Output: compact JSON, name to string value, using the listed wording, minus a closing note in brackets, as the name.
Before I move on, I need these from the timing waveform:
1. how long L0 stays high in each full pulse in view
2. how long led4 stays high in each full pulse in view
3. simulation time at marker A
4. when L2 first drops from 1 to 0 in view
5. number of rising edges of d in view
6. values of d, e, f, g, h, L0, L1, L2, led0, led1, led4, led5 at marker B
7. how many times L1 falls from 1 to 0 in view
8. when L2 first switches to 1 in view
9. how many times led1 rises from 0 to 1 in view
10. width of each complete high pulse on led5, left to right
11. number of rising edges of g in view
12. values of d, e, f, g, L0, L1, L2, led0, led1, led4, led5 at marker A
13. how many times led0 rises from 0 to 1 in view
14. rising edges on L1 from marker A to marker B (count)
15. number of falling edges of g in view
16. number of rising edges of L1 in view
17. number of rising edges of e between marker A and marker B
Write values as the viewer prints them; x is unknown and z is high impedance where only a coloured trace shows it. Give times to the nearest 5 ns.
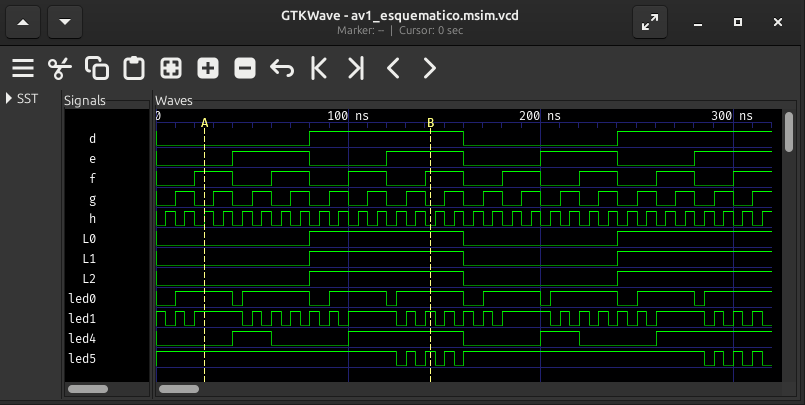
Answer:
{"how long L0 stays high in each full pulse in view": "80 ns", "how long led4 stays high in each full pulse in view": "20 ns, 60 ns, 20 ns", "simulation time at marker A": "25 ns", "when L2 first drops from 1 to 0 in view": "160 ns", "number of rising edges of d in view": "2", "values of d, e, f, g, h, L0, L1, L2, led0, led1, led4, led5 at marker B": "d=1, e=1, f=1, g=0, h=0, L0=1, L1=1, L2=1, led0=1, led1=1, led4=1, led5=1", "how many times L1 falls from 1 to 0 in view": "1", "when L2 first switches to 1 in view": "80 ns", "how many times led1 rises from 0 to 1 in view": "23", "width of each complete high pulse on led5, left to right": "5 ns, 5 ns, 5 ns, 125 ns, 5 ns, 5 ns, 5 ns", "number of rising edges of g in view": "16", "values of d, e, f, g, L0, L1, L2, led0, led1, led4, led5 at marker A": "d=0, e=0, f=1, g=0, L0=0, L1=0, L2=0, led0=1, led1=1, led4=0, led5=1", "how many times led0 rises from 0 to 1 in view": "8", "rising edges on L1 from marker A to marker B": "1", "number of falling edges of g in view": "15", "number of rising edges of L1 in view": "2", "number of rising edges of e between marker A and marker B": "2"}
